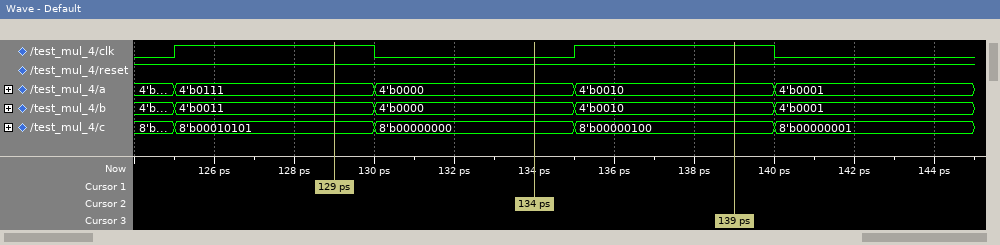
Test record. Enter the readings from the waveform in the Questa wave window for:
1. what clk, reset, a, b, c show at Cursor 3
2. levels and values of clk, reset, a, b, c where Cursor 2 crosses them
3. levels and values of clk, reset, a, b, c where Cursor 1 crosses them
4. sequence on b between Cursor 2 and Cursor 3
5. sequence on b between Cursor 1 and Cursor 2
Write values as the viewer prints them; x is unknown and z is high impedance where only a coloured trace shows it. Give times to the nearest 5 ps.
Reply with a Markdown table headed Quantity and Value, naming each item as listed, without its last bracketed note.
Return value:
| Quantity | Value |
|---|---|
| what clk, reset, a, b, c show at Cursor 3 | clk=1, reset=1, a=4'b0010, b=4'b0010, c=8'b00000100 |
| levels and values of clk, reset, a, b, c where Cursor 2 crosses them | clk=0, reset=1, a=4'b0000, b=4'b0000, c=8'b00000000 |
| levels and values of clk, reset, a, b, c where Cursor 1 crosses them | clk=1, reset=1, a=4'b0111, b=4'b0011, c=8'b00010101 |
| sequence on b between Cursor 2 and Cursor 3 | 4'b0000, 4'b0010 |
| sequence on b between Cursor 1 and Cursor 2 | 4'b0011, 4'b0000 |
